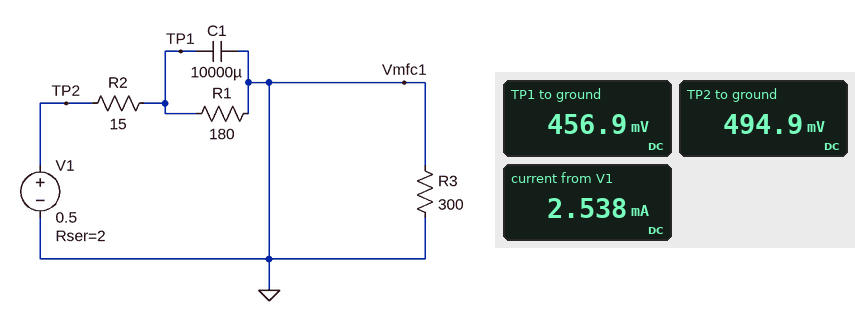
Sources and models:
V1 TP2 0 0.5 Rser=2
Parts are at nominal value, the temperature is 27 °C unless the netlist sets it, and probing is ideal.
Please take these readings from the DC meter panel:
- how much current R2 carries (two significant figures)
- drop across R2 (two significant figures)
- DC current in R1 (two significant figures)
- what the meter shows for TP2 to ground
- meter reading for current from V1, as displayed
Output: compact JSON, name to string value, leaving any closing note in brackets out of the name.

{"how much current R2 carries": "2.5 mA", "drop across R2": "38 mV", "DC current in R1": "2.5 mA", "what the meter shows for TP2 to ground": "494.9 mV", "meter reading for current from V1, as displayed": "2.538 mA"}
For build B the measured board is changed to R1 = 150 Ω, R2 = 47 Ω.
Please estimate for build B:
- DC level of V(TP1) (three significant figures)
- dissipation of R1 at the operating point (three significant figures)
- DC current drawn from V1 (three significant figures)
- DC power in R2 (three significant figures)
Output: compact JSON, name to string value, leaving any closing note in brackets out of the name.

{"DC level of V(TP1)": "377 mV", "dissipation of R1 at the operating point": "947 µW", "DC current drawn from V1": "2.51 mA", "DC power in R2": "297 µW"}
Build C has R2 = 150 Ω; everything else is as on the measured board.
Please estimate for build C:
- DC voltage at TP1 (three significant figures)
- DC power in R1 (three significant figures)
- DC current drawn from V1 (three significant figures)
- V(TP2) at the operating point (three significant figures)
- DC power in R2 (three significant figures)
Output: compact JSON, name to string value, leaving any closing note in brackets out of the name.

{"DC voltage at TP1": "271 mV", "DC power in R1": "408 µW", "DC current drawn from V1": "1.51 mA", "V(TP2) at the operating point": "497 mV", "DC power in R2": "340 µW"}
